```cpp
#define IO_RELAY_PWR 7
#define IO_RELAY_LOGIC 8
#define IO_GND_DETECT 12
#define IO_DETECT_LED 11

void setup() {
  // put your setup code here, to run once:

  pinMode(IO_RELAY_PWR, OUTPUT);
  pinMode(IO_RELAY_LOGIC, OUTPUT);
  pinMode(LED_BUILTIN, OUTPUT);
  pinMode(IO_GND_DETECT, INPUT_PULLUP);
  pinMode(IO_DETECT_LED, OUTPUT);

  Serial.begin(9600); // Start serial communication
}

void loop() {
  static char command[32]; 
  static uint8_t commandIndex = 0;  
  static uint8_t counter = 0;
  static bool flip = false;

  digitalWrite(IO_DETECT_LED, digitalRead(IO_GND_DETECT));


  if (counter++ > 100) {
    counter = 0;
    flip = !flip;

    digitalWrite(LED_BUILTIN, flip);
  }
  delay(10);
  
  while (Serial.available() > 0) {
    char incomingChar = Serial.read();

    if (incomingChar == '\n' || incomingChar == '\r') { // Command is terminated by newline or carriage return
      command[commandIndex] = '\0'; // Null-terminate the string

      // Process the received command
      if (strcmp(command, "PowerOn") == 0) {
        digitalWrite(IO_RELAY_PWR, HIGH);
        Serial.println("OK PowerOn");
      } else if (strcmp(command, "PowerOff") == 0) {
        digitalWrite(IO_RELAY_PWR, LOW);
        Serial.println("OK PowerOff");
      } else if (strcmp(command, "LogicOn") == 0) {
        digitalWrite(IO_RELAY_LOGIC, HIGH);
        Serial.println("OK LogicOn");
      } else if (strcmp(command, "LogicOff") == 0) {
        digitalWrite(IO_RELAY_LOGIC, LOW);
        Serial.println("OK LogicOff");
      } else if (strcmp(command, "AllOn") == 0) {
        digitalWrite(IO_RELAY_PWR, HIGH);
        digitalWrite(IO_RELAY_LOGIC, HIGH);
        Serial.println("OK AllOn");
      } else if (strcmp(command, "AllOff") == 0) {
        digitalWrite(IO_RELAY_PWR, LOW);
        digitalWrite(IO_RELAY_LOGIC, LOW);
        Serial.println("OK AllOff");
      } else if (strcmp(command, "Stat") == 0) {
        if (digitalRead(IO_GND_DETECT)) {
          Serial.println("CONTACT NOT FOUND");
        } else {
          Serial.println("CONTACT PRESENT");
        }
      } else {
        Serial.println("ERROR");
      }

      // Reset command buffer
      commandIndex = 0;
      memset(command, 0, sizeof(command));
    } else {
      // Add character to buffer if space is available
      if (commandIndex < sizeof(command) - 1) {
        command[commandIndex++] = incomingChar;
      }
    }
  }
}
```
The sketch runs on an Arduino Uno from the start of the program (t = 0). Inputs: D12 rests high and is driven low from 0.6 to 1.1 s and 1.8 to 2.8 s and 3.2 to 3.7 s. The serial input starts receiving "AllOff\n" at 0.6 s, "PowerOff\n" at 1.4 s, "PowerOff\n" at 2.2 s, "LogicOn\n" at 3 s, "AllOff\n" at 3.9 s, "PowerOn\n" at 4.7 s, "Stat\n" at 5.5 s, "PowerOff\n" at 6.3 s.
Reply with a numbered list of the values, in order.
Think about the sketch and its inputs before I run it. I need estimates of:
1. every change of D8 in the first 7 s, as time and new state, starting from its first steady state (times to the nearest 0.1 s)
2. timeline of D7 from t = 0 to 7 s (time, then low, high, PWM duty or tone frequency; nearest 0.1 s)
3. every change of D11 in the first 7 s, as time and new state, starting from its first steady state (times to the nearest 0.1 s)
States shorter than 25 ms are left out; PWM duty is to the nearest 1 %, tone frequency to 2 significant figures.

1. 0 s low; 3 s high; 3.9 s low
2. 0 s low; 4.7 s high; 6.3 s low
3. 0 s high; 0.6 s low; 1.1 s high; 1.8 s low; 2.8 s high; 3.2 s low; 3.7 s high
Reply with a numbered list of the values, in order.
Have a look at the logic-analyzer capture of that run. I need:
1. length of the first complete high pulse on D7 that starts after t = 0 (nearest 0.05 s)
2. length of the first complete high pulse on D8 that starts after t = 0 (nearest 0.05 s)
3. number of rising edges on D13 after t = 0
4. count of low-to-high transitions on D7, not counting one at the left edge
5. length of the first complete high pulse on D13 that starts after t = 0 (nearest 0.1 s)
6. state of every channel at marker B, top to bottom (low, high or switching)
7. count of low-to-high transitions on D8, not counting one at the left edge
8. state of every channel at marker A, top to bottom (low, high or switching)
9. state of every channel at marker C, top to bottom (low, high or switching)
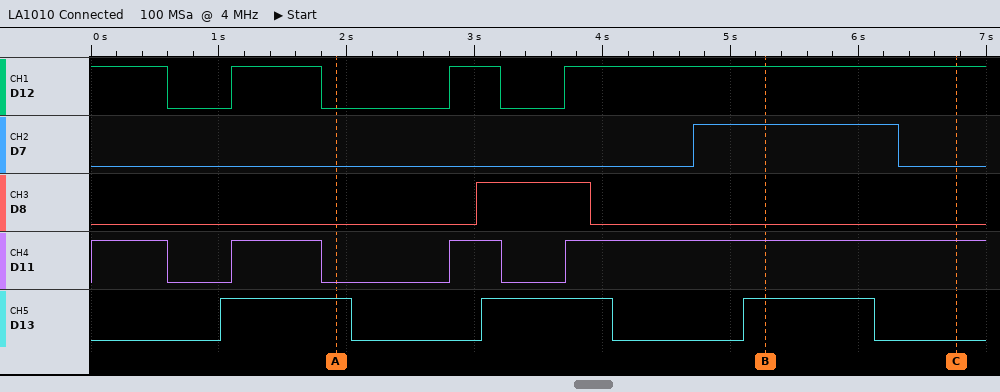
1. 1.60 s
2. 0.90 s
3. 3
4. 1
5. 1.0 s
6. D12 high, D7 high, D8 low, D11 high, D13 high
7. 1
8. D12 low, D7 low, D8 low, D11 low, D13 high
9. D12 high, D7 low, D8 low, D11 high, D13 low
